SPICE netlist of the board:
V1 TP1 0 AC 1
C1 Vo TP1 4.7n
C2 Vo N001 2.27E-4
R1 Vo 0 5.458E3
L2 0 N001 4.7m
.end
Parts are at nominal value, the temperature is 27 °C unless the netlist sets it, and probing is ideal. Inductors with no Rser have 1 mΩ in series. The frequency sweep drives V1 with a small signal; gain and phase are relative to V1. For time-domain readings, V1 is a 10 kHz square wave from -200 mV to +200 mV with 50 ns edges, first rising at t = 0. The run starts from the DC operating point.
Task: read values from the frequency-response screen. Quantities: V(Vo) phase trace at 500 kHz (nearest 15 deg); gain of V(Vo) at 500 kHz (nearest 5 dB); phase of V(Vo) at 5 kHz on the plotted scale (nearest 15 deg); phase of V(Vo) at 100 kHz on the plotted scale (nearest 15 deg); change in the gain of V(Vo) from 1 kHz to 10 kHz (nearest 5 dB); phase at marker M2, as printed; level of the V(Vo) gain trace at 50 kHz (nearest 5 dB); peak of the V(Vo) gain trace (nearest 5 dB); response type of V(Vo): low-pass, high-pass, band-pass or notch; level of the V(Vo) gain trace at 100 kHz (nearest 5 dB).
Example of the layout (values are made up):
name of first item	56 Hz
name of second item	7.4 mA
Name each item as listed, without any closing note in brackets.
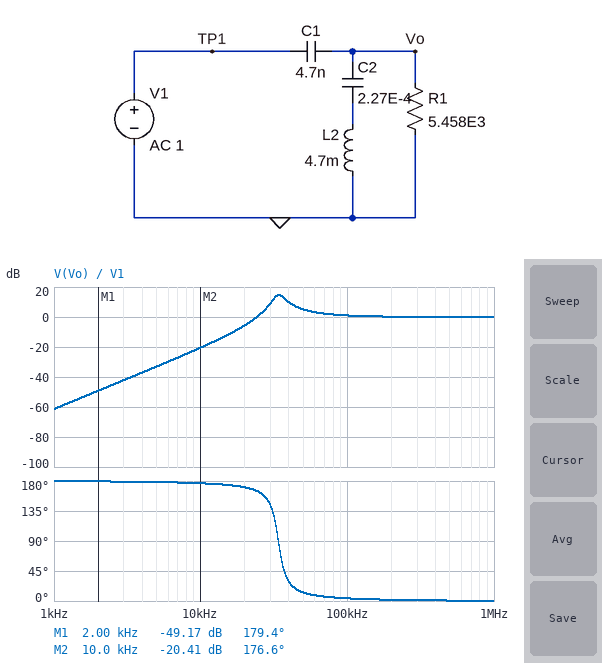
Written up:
V(Vo) phase trace at 500 kHz	0 deg
gain of V(Vo) at 500 kHz	0 dB
phase of V(Vo) at 5 kHz on the plotted scale	180 deg
phase of V(Vo) at 100 kHz on the plotted scale	0 deg
change in the gain of V(Vo) from 1 kHz to 10 kHz	40 dB
phase at marker M2, as printed	176.6 deg
level of the V(Vo) gain trace at 50 kHz	5 dB
peak of the V(Vo) gain trace	15 dB
response type of V(Vo): low-pass, high-pass, band-pass or notch	high-pass
level of the V(Vo) gain trace at 100 kHz	0 dB
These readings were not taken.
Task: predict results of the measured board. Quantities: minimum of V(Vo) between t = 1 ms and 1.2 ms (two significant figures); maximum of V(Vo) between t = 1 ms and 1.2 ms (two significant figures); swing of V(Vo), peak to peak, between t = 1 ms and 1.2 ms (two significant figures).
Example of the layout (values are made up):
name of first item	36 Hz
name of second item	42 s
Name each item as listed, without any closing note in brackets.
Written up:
minimum of V(Vo) between t = 1 ms and 1.2 ms	-390 mV
maximum of V(Vo) between t = 1 ms and 1.2 ms	390 mV
swing of V(Vo), peak to peak, between t = 1 ms and 1.2 ms	770 mV
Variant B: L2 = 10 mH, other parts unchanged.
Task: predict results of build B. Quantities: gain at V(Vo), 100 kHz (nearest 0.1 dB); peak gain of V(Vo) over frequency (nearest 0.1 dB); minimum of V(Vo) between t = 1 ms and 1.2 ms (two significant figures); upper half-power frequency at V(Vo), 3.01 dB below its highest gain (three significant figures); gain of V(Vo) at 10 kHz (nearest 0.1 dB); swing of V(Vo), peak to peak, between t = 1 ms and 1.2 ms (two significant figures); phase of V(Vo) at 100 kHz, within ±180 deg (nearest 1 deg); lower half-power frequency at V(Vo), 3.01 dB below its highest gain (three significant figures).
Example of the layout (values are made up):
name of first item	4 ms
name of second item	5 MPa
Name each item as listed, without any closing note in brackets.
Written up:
gain at V(Vo), 100 kHz	0.5 dB
peak gain of V(Vo) over frequency	11.5 dB
minimum of V(Vo) between t = 1 ms and 1.2 ms	-320 mV
upper half-power frequency at V(Vo), 3.01 dB below its highest gain	27.8 kHz
gain of V(Vo) at 10 kHz	-12.9 dB
swing of V(Vo), peak to peak, between t = 1 ms and 1.2 ms	640 mV
phase of V(Vo) at 100 kHz, within ±180 deg	4 deg
lower half-power frequency at V(Vo), 3.01 dB below its highest gain	20.9 kHz
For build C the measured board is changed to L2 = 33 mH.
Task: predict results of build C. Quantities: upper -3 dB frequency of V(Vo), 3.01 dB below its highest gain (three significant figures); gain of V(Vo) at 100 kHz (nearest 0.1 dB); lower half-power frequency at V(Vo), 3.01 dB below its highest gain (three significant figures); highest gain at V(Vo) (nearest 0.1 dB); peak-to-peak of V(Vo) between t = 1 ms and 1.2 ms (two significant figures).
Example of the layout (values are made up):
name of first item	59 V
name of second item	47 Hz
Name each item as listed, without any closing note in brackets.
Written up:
upper -3 dB frequency of V(Vo), 3.01 dB below its highest gain	19.9 kHz
gain of V(Vo) at 100 kHz	0.1 dB
lower half-power frequency at V(Vo), 3.01 dB below its highest gain	11.0 kHz
highest gain at V(Vo)	6.5 dB
peak-to-peak of V(Vo) between t = 1 ms and 1.2 ms	890 mV
